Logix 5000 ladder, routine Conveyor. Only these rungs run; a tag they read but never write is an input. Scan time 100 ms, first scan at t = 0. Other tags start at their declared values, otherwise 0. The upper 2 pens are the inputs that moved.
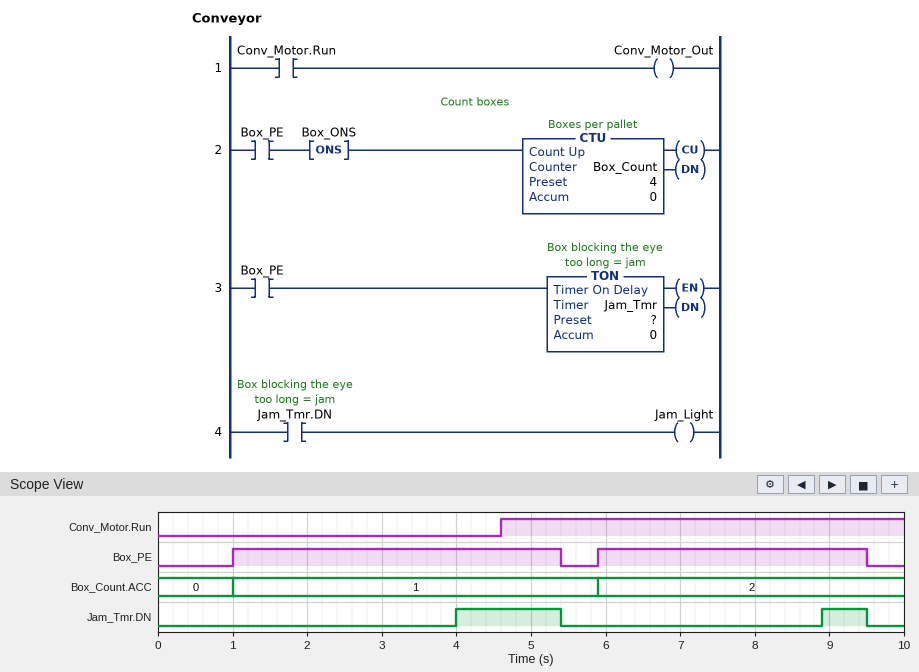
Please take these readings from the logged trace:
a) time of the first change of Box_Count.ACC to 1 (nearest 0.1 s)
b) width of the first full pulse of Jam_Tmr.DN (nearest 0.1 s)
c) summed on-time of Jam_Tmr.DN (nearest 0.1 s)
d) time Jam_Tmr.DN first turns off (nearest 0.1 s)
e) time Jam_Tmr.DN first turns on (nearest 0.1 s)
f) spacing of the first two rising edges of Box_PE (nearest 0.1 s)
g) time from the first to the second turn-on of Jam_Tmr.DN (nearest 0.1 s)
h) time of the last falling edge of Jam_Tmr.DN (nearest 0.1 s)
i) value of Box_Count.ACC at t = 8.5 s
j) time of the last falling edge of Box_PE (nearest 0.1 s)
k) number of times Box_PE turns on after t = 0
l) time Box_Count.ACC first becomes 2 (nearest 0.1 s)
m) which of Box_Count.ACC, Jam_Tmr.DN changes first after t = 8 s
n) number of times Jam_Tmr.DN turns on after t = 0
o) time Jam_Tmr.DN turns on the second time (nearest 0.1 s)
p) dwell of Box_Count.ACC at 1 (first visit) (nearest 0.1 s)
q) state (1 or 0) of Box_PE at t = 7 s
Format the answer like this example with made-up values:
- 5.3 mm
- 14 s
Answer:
- 1.0 s
- 1.4 s
- 2.0 s
- 5.4 s
- 4.0 s
- 4.9 s
- 4.9 s
- 9.5 s
- 2
- 9.5 s
- 2
- 5.9 s
- Jam_Tmr.DN
- 2
- 8.9 s
- 4.9 s
- 1
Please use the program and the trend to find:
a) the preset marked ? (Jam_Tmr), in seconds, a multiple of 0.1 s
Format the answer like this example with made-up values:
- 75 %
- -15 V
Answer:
- 3.0 s
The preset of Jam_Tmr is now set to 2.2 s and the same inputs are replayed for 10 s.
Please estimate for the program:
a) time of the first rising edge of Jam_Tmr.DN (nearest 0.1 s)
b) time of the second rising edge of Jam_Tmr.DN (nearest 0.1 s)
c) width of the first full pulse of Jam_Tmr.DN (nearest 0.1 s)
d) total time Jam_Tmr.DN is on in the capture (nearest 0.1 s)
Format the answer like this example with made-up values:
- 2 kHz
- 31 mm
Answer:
- 3.2 s
- 8.1 s
- 2.2 s
- 3.6 s
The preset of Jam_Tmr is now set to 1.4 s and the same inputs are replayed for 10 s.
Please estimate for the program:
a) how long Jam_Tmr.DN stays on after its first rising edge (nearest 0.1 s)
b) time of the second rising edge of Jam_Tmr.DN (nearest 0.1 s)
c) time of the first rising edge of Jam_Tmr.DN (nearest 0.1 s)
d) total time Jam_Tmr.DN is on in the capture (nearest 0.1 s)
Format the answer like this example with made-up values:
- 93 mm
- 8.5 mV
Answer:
- 3.0 s
- 7.3 s
- 2.4 s
- 5.2 s
